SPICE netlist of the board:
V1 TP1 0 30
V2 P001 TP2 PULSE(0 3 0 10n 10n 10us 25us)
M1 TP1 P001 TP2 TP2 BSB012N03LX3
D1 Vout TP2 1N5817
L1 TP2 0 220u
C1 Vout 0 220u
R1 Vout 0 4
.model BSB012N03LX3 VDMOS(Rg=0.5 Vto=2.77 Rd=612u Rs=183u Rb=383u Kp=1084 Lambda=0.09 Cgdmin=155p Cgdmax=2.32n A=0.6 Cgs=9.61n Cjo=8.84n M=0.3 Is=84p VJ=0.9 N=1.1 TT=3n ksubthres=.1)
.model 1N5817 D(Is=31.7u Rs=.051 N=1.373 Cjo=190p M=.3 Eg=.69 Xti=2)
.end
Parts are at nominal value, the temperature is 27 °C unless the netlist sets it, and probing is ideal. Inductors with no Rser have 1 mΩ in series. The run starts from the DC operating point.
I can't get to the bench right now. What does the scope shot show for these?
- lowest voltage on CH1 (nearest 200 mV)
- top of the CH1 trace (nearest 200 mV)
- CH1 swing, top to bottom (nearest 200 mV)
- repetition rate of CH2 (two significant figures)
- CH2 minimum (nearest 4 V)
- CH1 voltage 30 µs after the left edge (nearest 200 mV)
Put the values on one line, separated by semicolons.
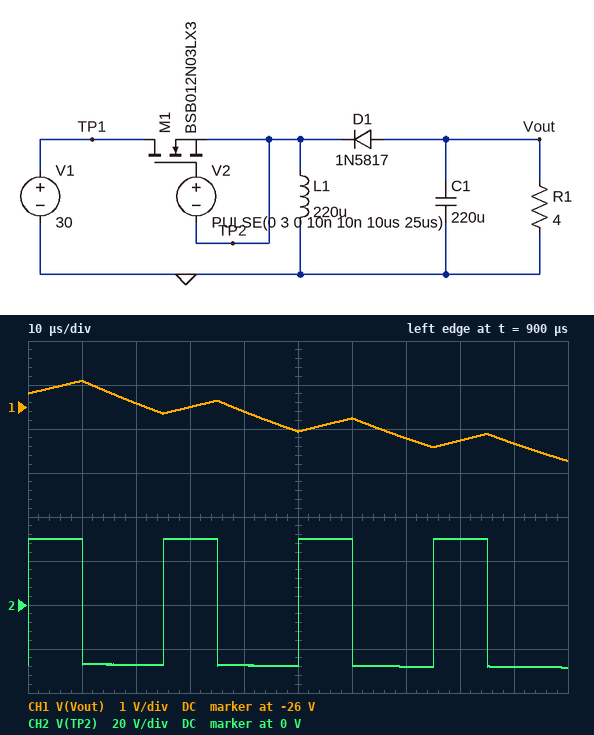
-27.2 V; -25.4 V; 1.8 V; 40 kHz; -28 V; -26.0 V
